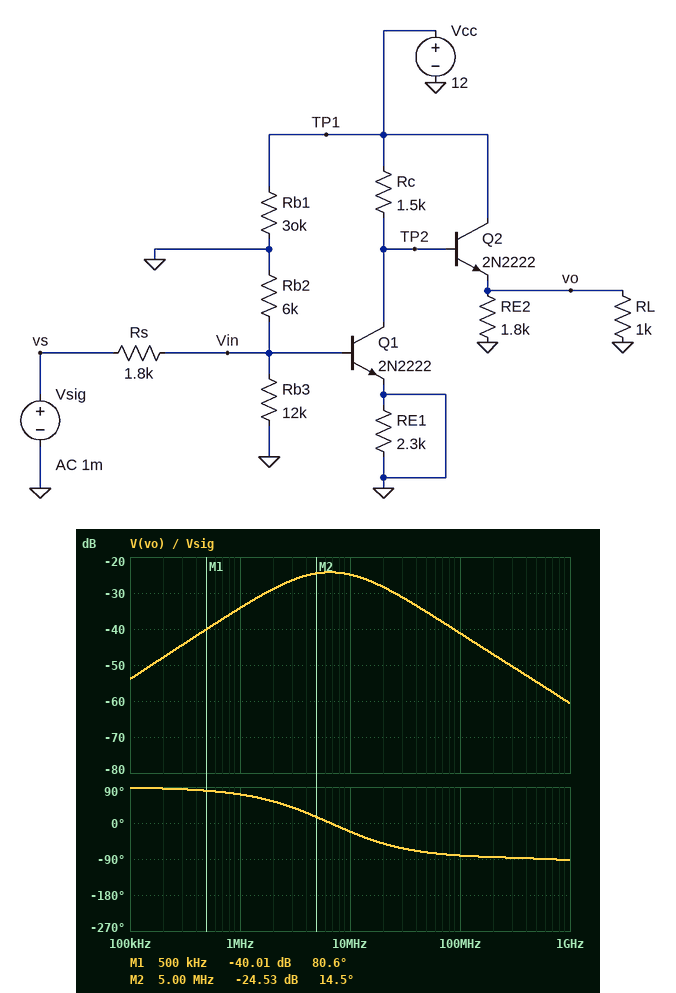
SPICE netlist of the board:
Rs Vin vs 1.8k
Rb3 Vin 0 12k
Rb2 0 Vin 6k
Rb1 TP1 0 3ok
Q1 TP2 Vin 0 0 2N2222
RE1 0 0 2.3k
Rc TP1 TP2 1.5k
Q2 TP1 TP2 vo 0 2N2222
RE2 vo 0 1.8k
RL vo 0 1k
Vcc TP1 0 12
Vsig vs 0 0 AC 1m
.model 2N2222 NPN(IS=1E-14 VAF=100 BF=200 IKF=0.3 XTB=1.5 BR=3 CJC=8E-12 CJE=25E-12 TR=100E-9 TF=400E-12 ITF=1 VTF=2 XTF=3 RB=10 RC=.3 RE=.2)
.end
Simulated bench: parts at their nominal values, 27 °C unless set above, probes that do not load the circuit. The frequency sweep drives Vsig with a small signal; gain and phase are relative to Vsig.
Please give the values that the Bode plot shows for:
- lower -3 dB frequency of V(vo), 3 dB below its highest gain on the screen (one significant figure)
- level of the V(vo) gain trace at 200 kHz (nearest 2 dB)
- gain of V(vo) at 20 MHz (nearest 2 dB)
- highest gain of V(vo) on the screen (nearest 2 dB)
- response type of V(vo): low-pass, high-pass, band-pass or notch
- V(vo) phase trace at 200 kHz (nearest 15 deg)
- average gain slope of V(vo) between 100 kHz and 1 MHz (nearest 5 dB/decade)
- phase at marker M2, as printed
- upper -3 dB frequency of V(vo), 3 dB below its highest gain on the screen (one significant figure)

3 MHz
-48 dB
-28 dB
-24 dB
band-pass
90 deg
20 dB/decade
14.5 deg
20 MHz
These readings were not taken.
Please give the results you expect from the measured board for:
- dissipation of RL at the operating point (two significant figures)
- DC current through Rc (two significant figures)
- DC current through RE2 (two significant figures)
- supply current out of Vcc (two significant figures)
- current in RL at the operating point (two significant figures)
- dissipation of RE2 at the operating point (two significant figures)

120 mW
91 µA
6.2 mA
4.0 A
11 mA
69 mW
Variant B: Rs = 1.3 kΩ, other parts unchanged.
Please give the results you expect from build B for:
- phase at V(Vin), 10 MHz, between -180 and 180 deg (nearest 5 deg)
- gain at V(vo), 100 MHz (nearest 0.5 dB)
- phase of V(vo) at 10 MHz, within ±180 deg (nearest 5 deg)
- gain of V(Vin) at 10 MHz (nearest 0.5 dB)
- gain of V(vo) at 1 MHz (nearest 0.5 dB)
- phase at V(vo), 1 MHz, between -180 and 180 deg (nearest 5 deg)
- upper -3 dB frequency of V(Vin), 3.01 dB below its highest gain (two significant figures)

-60 deg
-38.5 dB
-15 deg
-8.5 dB
-33.5 dB
75 deg
5.7 MHz
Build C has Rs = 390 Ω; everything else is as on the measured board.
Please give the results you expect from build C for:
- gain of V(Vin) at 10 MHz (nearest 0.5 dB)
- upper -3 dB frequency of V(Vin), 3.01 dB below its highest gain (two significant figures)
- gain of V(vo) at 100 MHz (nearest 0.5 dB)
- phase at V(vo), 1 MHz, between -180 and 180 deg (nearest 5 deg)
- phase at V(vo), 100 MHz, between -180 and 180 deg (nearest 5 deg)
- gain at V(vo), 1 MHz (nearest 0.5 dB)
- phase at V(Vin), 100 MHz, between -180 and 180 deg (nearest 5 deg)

-2.5 dB
16 MHz
-28.0 dB
80 deg
-75 deg
-31.5 dB
-70 deg
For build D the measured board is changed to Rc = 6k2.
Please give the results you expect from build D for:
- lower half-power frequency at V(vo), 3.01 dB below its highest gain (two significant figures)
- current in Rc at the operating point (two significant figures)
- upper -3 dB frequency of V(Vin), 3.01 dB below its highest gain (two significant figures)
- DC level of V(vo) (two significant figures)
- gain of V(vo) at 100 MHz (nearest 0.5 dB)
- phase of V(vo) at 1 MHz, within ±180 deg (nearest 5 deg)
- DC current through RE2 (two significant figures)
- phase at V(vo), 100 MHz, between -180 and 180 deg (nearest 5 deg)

1.4 MHz
87 µA
4.6 MHz
11 V
-40.5 dB
55 deg
6.0 mA
-85 deg
